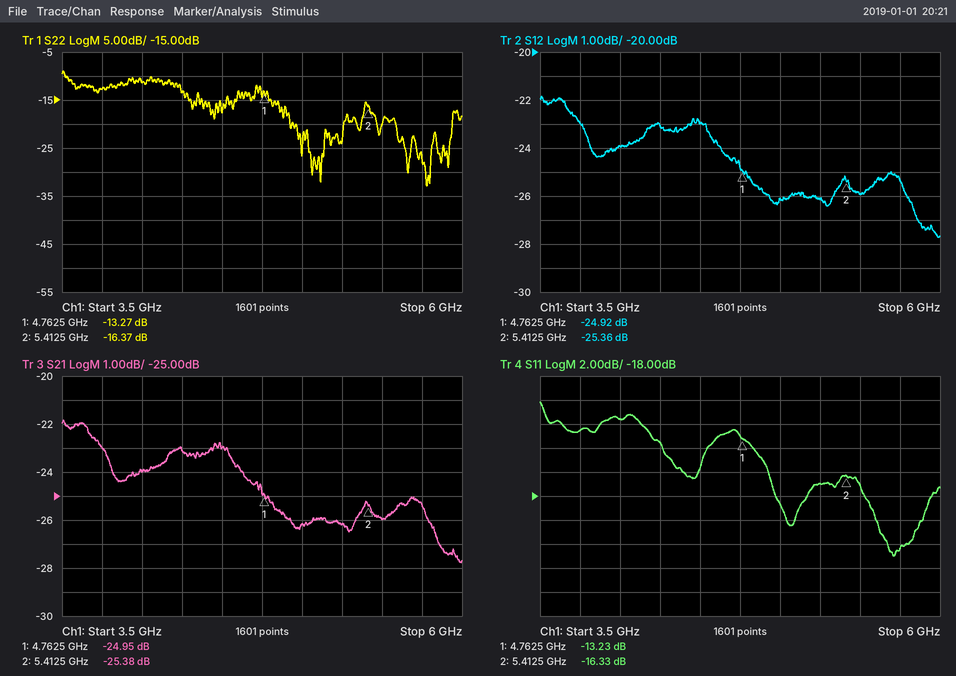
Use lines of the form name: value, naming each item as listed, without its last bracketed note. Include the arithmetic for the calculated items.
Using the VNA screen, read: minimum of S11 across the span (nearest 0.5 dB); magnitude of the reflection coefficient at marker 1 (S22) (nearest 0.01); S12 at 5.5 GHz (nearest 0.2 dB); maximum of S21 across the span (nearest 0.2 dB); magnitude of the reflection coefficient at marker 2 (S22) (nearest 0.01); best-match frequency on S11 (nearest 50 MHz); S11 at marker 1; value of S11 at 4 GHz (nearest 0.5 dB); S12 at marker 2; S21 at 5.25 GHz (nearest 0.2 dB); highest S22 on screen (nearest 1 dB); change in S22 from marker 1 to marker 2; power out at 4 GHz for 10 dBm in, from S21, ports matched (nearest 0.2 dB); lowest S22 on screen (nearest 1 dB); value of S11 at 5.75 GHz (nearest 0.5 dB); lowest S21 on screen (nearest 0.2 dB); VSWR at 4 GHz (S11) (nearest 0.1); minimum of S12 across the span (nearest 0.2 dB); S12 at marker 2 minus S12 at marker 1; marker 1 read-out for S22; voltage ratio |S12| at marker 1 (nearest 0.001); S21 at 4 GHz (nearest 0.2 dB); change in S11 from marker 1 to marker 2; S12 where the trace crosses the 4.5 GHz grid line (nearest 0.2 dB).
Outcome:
minimum of S11 across the span: -23.0 dB
magnitude of the reflection coefficient at marker 1 (S22): 10^(-13.27/20) ≈ 0.22
S12 at 5.5 GHz: -26.0 dB
maximum of S21 across the span: -21.8 dB
magnitude of the reflection coefficient at marker 2 (S22): 10^(-16.37/20) ≈ 0.15
best-match frequency on S11: 5.70 GHz
S11 at marker 1: -13.23 dB
value of S11 at 4 GHz: -11.5 dB
S12 at marker 2: -25.36 dB
S21 at 5.25 GHz: -26.2 dB
highest S22 on screen: -9 dB
change in S22 from marker 1 to marker 2: -16.37 − (-13.27) = -3.10 dB
power out at 4 GHz for 10 dBm in, from S21, ports matched: 10 dBm + (-24.0 dB) = -14.0 dBm
lowest S22 on screen: -33 dB
value of S11 at 5.75 GHz: -22.5 dB
lowest S21 on screen: -27.8 dB
VSWR at 4 GHz (S11): |Γ| = 10^(-11.5/20) = 0.2661; VSWR = (1 + 0.2661)/(1 − 0.2661) ≈ 1.7
minimum of S12 across the span: -27.8 dB
S12 at marker 2 minus S12 at marker 1: -25.36 − (-24.92) = -0.44 dB
marker 1 read-out for S22: -13.27 dB
voltage ratio |S12| at marker 1: 10^(-24.92/20) ≈ 0.057
S21 at 4 GHz: -24.0 dB
change in S11 from marker 1 to marker 2: -16.33 − (-13.23) = -3.10 dB
S12 where the trace crosses the 4.5 GHz grid line: -23.0 dB
